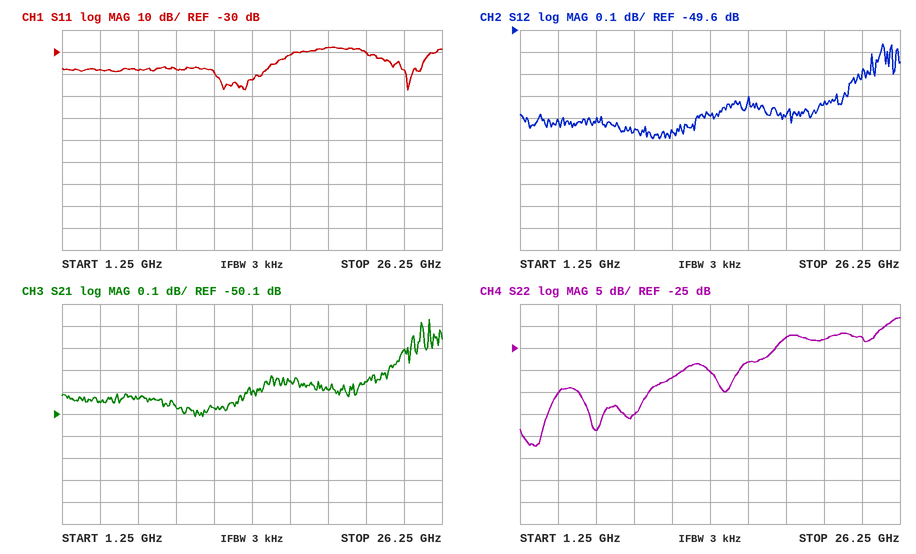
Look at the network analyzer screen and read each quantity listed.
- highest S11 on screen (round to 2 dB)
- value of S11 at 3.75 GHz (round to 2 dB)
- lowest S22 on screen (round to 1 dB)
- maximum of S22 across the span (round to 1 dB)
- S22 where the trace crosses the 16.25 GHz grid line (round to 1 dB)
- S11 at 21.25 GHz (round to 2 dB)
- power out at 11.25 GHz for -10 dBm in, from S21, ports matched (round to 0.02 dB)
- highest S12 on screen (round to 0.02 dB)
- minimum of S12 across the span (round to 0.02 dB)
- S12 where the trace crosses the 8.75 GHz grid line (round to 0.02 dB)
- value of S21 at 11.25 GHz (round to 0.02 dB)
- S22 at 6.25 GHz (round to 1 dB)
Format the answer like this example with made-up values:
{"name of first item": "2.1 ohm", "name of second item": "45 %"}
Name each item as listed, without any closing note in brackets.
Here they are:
{"highest S11 on screen": "-28 dB", "value of S11 at 3.75 GHz": "-38 dB", "lowest S22 on screen": "-47 dB", "maximum of S22 across the span": "-18 dB", "S22 where the trace crosses the 16.25 GHz grid line": "-28 dB", "S11 at 21.25 GHz": "-30 dB", "power out at 11.25 GHz for -10 dBm in, from S21, ports matched": "-60.08 dBm", "highest S12 on screen": "-49.66 dB", "minimum of S12 across the span": "-50.10 dB", "S12 where the trace crosses the 8.75 GHz grid line": "-50.06 dB", "value of S21 at 11.25 GHz": "-50.08 dB", "S22 at 6.25 GHz": "-44 dB"}
